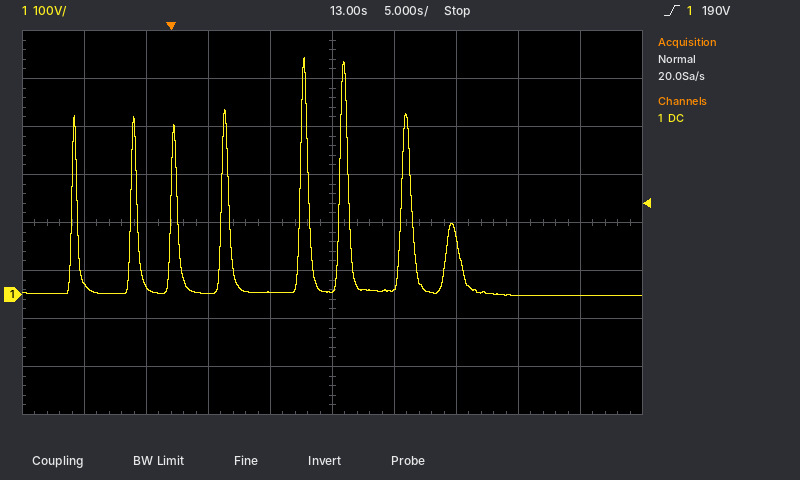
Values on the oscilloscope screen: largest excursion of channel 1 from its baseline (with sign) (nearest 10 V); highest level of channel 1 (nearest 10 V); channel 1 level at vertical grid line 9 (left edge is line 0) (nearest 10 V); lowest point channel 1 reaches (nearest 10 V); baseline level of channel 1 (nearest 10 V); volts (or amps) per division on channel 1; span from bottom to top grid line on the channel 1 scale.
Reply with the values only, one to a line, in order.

+490 V
490 V
0 V
0 V
0 V
100 V
800 V
